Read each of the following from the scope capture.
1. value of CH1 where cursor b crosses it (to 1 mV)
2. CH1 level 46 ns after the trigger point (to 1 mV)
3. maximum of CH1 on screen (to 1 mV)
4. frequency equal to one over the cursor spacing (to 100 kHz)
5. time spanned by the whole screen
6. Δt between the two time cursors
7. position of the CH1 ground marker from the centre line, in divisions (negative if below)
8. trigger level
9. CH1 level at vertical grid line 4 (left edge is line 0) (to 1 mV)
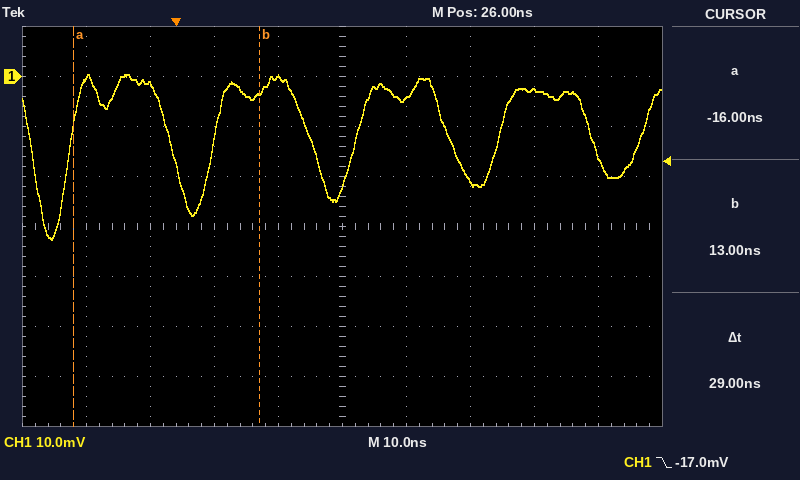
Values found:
-3 mV
-21 mV
0 mV
34.5 MHz
100 ns
29 ns
+3.0 div
-17.0 mV
0 mV
